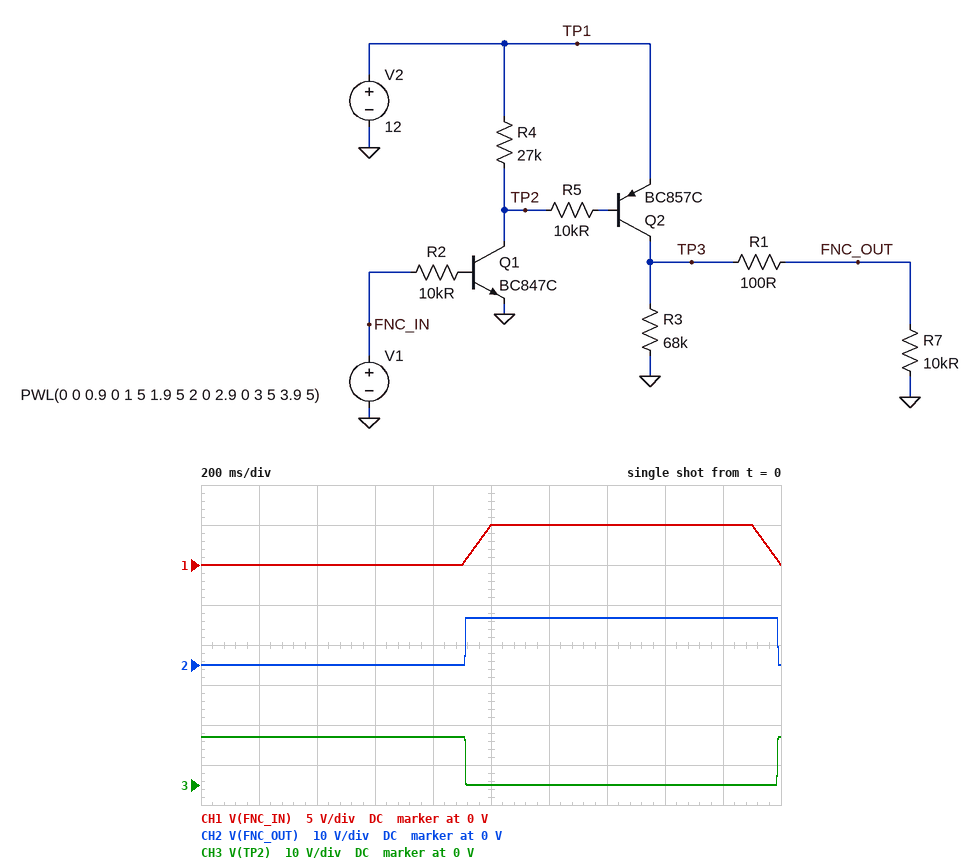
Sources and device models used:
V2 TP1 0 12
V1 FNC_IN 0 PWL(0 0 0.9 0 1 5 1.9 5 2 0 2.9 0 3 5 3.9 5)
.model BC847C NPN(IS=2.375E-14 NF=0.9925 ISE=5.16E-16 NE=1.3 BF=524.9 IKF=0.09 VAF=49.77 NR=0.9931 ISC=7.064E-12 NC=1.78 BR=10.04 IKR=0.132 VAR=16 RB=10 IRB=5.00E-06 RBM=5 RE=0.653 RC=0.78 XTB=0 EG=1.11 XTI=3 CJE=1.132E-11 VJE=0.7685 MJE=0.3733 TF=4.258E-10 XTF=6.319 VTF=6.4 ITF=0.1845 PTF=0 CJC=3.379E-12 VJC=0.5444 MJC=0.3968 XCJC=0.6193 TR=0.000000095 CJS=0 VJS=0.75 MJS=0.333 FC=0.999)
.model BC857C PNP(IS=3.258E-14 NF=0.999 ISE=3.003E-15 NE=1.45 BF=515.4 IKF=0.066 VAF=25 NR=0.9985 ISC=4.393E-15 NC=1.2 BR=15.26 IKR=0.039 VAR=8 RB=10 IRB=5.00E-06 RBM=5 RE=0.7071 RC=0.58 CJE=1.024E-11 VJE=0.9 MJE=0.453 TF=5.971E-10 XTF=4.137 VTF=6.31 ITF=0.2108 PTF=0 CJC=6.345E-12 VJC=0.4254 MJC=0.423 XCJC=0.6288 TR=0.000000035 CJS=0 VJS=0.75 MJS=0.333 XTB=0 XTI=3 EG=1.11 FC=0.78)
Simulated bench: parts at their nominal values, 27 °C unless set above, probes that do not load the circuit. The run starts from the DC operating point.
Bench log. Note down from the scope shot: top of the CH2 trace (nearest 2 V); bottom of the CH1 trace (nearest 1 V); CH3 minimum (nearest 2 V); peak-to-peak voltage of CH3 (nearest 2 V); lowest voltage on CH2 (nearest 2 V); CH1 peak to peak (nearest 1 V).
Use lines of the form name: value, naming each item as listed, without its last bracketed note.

top of the CH2 trace: 12 V
bottom of the CH1 trace: 0 V
CH3 minimum: 0 V
peak-to-peak voltage of CH3: 12 V
lowest voltage on CH2: 0 V
CH1 peak to peak: 5 V
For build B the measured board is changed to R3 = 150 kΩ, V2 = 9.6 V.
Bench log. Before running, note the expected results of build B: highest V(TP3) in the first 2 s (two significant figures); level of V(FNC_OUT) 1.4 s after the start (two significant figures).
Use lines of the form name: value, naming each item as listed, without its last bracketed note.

highest V(TP3) in the first 2 s: 9.6 V
level of V(FNC_OUT) 1.4 s after the start: 9.5 V
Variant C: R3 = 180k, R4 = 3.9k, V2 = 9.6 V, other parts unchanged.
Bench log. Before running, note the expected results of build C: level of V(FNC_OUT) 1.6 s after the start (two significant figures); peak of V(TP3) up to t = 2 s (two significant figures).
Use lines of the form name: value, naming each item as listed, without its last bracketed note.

level of V(FNC_OUT) 1.6 s after the start: 9.5 V
peak of V(TP3) up to t = 2 s: 9.6 V
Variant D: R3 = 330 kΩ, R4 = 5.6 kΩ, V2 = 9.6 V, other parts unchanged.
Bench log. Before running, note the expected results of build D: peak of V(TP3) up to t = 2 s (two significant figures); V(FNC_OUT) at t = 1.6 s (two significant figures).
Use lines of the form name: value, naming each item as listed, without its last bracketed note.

peak of V(TP3) up to t = 2 s: 9.6 V
V(FNC_OUT) at t = 1.6 s: 9.5 V
